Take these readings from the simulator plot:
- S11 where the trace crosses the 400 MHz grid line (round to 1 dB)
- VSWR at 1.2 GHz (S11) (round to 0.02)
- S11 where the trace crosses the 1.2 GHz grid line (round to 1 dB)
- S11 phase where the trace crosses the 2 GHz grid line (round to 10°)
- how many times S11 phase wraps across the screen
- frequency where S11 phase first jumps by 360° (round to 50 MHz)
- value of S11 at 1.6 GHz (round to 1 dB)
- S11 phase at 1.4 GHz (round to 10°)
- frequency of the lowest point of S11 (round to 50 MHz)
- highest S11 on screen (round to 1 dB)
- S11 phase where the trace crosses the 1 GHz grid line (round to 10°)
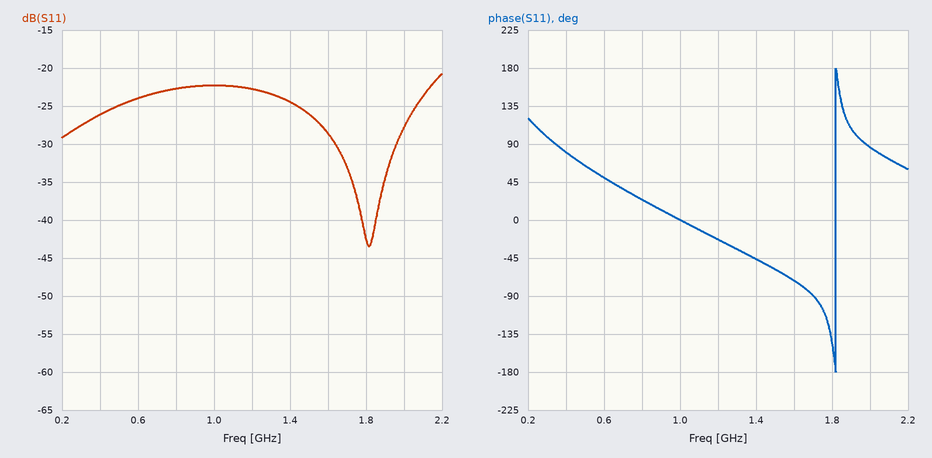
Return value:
-26 dB
1.16
-23 dB
90°
1
1.80 GHz
-29 dB
-50°
1.80 GHz
-21 dB
0°
